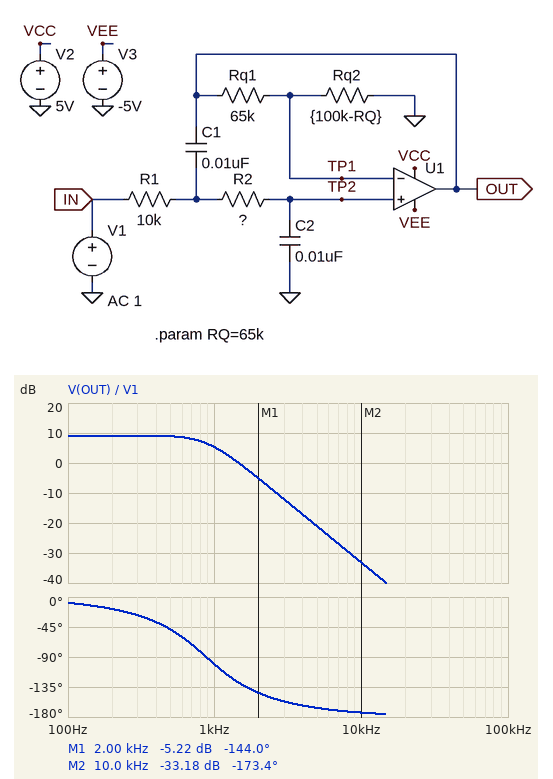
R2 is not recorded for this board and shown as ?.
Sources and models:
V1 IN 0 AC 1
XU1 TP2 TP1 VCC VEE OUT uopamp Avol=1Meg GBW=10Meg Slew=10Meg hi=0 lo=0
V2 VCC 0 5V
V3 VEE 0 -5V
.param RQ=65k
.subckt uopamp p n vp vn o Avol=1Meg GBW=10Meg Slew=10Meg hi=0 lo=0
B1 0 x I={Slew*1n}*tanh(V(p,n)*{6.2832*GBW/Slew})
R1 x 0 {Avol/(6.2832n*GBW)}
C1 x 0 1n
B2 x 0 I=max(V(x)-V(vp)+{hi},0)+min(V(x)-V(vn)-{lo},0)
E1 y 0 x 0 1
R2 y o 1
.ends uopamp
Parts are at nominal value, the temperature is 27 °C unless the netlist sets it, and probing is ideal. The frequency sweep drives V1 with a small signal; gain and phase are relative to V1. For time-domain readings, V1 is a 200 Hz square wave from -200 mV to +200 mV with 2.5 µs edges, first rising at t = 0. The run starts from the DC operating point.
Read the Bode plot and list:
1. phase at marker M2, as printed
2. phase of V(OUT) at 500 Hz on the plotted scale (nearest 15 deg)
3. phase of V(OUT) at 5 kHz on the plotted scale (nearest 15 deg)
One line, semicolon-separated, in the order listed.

-173.4 deg; -45 deg; -165 deg
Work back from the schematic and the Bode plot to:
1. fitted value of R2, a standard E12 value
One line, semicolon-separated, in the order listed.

33 kΩ
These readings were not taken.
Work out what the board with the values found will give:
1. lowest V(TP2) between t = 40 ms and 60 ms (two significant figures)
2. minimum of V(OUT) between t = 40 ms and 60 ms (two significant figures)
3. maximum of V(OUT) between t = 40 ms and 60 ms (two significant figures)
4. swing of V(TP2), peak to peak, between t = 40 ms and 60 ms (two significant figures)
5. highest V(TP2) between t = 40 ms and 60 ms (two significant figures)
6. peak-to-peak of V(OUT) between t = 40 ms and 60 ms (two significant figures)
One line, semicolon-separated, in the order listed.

-220 mV; -640 mV; 640 mV; 450 mV; 220 mV; 1.3 V
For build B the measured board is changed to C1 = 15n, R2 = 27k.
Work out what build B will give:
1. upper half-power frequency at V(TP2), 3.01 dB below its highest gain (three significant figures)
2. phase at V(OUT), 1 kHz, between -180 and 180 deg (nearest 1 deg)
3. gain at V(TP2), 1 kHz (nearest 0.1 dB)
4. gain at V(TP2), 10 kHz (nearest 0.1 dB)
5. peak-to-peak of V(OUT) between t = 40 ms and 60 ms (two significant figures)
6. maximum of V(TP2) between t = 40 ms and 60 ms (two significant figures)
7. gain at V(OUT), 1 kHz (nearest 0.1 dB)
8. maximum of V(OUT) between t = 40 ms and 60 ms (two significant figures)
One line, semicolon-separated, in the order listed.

915 Hz; -136 deg; 1.6 dB; -44.0 dB; 2.2 V; 380 mV; 10.7 dB; 1.1 V
